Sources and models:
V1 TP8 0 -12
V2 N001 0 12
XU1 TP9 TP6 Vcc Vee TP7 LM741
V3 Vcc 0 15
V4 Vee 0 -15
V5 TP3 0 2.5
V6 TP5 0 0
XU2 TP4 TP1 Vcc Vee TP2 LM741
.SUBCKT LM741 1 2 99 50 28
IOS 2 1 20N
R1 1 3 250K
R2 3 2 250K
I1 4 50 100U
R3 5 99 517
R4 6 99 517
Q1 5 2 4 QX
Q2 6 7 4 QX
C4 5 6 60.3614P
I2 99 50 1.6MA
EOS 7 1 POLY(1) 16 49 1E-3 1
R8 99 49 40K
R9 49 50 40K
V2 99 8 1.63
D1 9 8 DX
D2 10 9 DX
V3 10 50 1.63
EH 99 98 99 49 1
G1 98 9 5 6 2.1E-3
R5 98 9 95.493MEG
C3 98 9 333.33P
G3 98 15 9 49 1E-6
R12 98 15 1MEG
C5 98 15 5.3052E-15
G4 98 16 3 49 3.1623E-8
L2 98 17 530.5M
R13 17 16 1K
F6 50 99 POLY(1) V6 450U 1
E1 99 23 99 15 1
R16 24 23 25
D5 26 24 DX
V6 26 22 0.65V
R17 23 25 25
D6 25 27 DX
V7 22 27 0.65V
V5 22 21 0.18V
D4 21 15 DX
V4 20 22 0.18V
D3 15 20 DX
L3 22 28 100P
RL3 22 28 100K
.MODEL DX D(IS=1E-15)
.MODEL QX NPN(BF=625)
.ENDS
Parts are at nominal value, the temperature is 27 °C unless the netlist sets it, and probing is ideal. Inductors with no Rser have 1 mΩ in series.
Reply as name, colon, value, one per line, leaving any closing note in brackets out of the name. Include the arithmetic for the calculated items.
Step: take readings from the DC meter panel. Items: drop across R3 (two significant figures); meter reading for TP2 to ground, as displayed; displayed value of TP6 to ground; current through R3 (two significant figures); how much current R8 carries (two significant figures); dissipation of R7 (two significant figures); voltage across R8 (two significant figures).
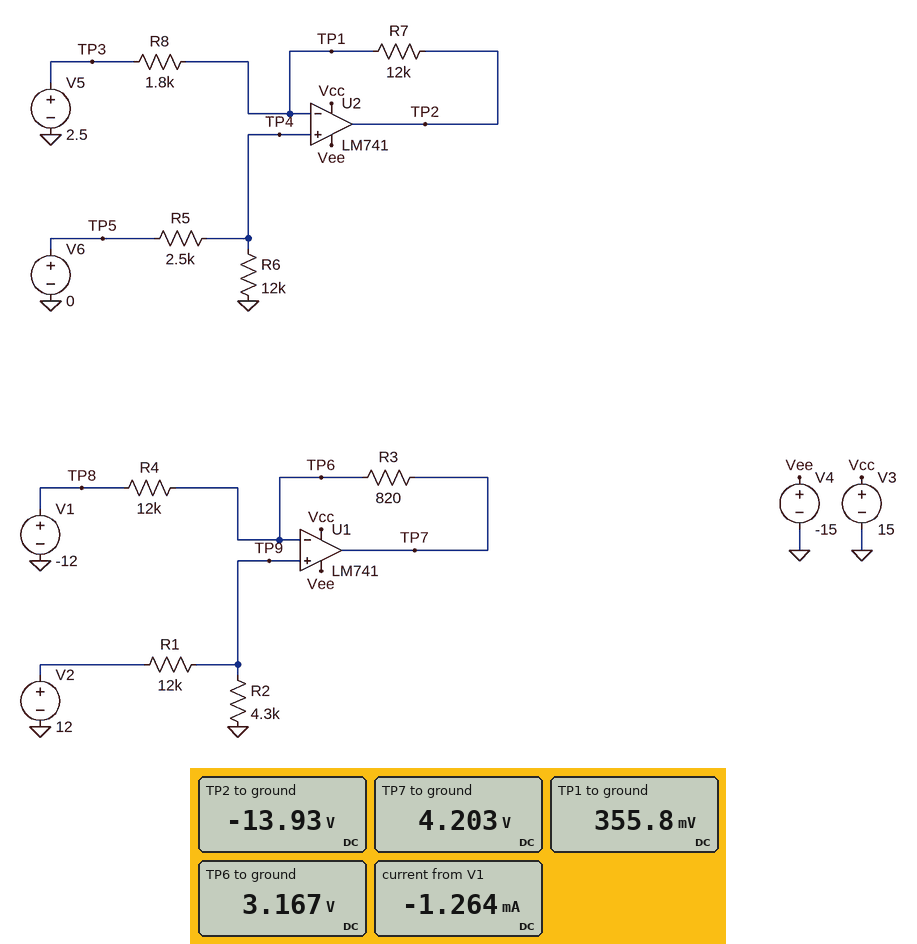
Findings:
drop across R3: 4.203 V - 3.167 V = 1.0 V
meter reading for TP2 to ground, as displayed: -13.93 V
displayed value of TP6 to ground: 3.167 V
current through R3: (4.203 V - 3.167 V) / 820 Ω = 1.3 mA
how much current R8 carries: (2.5 V - 355.8 mV) / 1.8 kΩ = 1.2 mA
dissipation of R7: (355.8 mV - (-13.93 V))^2 / 12 kΩ = 17 mW
voltage across R8: 2.5 V - 355.8 mV = 2.1 V
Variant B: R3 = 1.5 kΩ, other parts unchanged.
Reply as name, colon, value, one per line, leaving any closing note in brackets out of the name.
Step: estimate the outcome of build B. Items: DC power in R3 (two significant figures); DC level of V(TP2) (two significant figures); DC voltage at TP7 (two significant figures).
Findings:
DC power in R3: 2.4 mW
DC level of V(TP2): -14 V
DC voltage at TP7: 5.1 V
